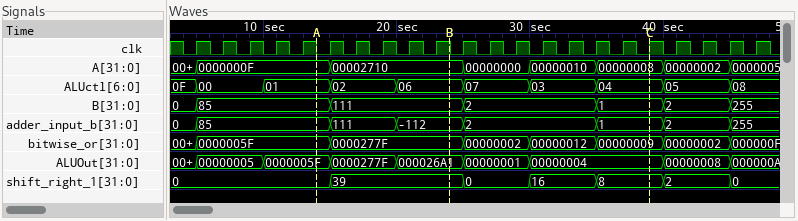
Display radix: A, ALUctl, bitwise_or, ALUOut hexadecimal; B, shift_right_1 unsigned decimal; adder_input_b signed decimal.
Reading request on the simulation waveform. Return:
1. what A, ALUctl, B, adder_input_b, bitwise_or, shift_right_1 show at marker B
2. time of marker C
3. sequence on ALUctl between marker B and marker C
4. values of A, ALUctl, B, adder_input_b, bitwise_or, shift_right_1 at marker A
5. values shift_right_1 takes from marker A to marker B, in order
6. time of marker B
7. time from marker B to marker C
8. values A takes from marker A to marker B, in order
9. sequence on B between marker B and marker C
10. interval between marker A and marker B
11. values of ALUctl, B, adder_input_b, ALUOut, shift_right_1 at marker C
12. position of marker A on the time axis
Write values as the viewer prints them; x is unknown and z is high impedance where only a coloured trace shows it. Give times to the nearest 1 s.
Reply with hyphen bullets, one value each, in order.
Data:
- A=00002710, ALUctl=06, B=111, adder_input_b=-112, bitwise_or=0000277F, shift_right_1=39
- 39 s
- 06, 07, 03, 04
- A=0000000F, ALUctl=01, B=85, adder_input_b=85, bitwise_or=0000005F, shift_right_1=0
- 0, 39
- 24 s
- 15 s
- 0000000F, 00002710
- 111, 2, 1
- 10 s
- ALUctl=04, B=1, adder_input_b=1, ALUOut=00000004, shift_right_1=8
- 14 s
